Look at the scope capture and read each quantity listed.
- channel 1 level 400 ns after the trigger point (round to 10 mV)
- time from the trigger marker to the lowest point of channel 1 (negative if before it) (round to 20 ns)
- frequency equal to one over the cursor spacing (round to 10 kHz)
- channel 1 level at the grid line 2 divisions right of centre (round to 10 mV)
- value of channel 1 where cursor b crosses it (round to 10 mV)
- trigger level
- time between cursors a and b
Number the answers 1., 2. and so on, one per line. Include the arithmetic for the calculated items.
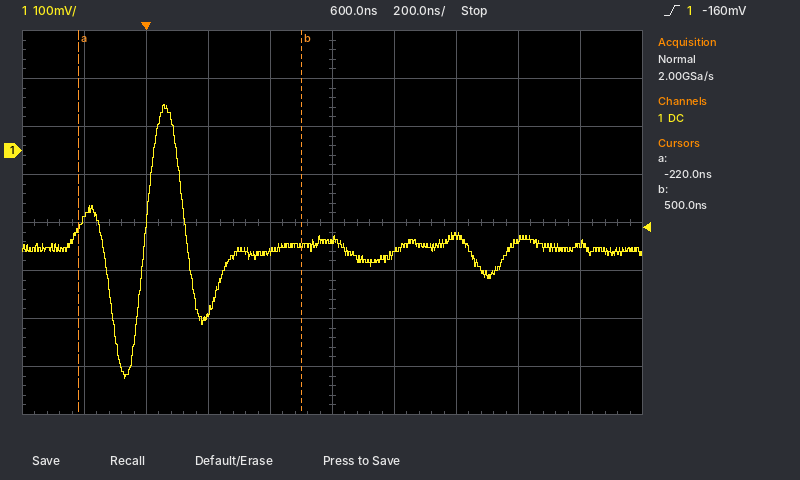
1. -210 mV
2. -60 ns
3. 1 / 720 ns ≈ 1.39 MHz
4. -180 mV
5. -200 mV
6. -160 mV
7. 500 ns − (-220 ns) = 720 ns
